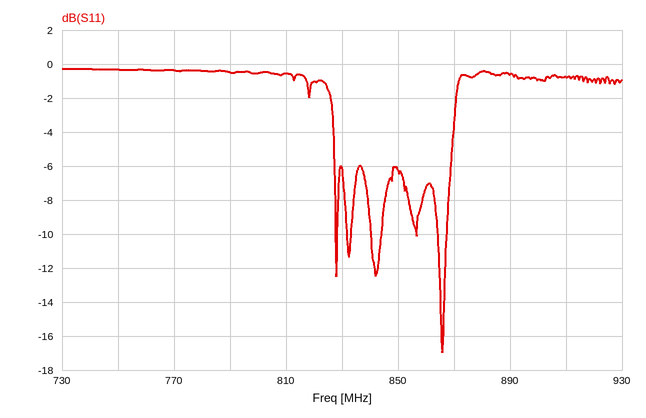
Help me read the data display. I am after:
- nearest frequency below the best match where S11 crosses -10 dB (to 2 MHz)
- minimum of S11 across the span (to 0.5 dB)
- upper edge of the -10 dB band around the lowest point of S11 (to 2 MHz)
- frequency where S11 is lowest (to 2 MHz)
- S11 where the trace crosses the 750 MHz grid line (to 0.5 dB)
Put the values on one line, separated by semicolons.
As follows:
864 MHz; -17.0 dB; 868 MHz; 866 MHz; -0.5 dB
